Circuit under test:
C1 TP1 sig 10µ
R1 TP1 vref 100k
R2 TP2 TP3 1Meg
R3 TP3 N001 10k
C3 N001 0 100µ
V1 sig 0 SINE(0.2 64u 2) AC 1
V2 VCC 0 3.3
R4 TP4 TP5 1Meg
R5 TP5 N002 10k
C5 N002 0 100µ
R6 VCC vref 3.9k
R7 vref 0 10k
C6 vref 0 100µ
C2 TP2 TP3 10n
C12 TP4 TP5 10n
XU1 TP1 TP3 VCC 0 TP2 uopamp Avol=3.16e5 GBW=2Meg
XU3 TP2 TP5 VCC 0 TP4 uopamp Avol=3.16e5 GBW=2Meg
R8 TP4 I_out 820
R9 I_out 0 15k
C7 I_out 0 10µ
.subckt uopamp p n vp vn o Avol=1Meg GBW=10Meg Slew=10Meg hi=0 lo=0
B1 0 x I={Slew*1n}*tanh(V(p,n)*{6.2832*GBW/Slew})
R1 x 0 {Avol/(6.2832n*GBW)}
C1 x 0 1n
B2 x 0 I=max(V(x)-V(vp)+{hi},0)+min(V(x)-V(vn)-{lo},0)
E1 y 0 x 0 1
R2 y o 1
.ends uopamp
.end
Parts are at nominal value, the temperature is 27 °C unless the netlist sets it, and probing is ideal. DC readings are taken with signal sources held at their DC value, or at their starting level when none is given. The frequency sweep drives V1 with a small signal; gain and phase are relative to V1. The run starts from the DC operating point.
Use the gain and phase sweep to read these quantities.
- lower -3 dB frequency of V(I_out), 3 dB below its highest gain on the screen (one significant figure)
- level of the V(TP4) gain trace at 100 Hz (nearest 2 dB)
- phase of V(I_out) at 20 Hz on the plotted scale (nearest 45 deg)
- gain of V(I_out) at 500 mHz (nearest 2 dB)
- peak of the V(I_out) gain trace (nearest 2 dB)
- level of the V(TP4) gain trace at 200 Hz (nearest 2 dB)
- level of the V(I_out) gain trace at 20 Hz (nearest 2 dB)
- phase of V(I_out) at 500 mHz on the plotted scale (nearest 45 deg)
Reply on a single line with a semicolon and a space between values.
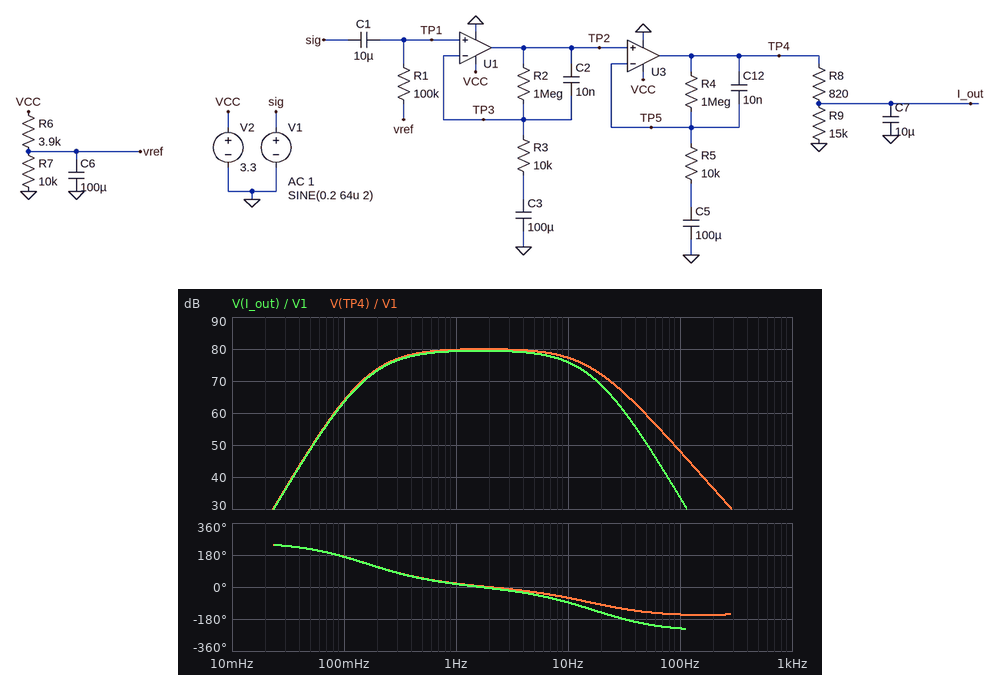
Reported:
300 mHz; 48 dB; -135 deg; 78 dB; 80 dB; 36 dB; 68 dB; 45 deg
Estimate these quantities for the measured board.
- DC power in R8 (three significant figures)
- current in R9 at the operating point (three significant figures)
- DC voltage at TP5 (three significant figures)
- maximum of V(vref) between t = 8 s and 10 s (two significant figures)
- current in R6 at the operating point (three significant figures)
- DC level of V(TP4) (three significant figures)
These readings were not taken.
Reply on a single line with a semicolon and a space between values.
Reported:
18.5 µW; 150 µA; 2.37 V; 2.4 V; 237 µA; 2.37 V
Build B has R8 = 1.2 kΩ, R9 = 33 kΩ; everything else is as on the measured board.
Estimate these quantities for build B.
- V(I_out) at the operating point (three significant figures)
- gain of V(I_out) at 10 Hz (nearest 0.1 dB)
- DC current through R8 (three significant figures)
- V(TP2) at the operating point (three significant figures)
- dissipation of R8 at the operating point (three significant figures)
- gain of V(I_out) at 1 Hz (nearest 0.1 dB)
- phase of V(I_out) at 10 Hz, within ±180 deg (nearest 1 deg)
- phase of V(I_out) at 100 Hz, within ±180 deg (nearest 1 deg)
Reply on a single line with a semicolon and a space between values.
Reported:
2.29 V; 75.1 dB; 69.4 µA; 2.37 V; 5.78 µW; 79.5 dB; -97 deg; 123 deg
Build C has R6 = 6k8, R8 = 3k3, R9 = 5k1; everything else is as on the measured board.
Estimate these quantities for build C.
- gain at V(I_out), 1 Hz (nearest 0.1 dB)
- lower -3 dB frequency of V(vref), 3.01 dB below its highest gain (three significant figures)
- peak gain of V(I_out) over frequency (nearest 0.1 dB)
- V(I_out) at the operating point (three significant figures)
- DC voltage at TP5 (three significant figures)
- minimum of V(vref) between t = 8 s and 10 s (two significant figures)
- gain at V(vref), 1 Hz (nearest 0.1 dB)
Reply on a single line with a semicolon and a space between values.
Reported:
75.4 dB; 94.4 mHz; 75.5 dB; 1.19 V; 1.96 V; 2.0 V; -36.8 dB
